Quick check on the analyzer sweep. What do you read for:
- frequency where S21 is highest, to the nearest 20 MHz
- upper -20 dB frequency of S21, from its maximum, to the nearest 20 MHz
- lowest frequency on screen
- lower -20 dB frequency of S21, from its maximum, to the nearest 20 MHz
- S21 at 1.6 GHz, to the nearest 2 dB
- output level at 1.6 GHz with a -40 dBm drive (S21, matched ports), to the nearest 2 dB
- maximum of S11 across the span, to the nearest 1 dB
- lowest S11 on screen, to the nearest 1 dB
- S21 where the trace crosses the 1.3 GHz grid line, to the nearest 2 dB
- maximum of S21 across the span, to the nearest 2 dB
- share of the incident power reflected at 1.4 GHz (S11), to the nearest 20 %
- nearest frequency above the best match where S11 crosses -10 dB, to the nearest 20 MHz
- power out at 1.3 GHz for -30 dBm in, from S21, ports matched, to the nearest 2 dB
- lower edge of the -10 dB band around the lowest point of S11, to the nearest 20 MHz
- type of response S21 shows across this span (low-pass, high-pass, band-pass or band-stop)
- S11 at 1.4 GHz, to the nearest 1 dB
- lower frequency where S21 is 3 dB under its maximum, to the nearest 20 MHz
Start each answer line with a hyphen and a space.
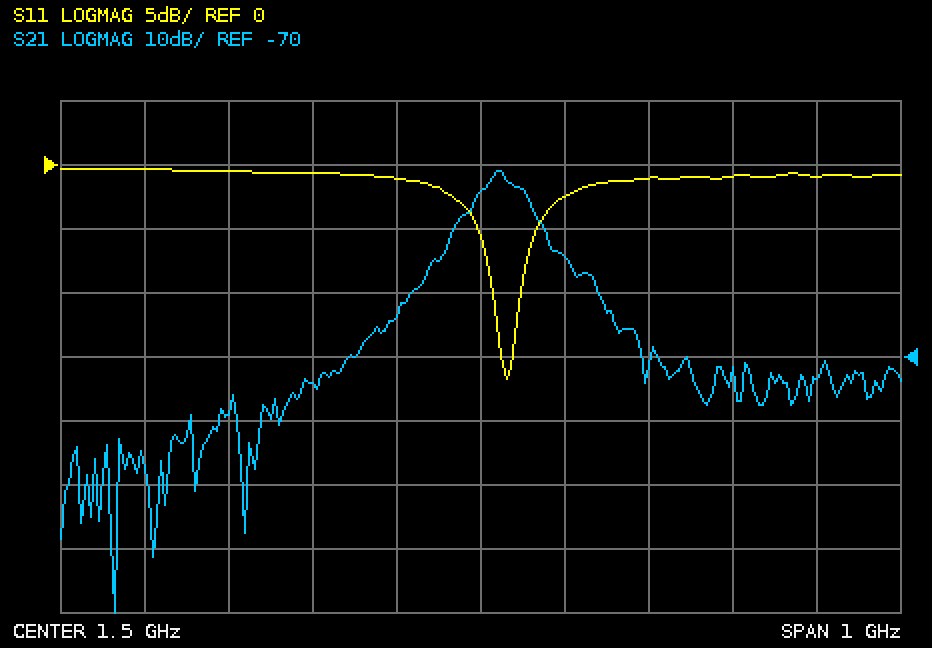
- 1.52 GHz
- 1.64 GHz
- 1 GHz
- 1.42 GHz
- -54 dB
- -94 dBm
- 0 dB
- -17 dB
- -74 dB
- -40 dB
- 80 %
- 1.54 GHz
- -104 dBm
- 1.52 GHz
- band-pass
- -1 dB
- 1.50 GHz
